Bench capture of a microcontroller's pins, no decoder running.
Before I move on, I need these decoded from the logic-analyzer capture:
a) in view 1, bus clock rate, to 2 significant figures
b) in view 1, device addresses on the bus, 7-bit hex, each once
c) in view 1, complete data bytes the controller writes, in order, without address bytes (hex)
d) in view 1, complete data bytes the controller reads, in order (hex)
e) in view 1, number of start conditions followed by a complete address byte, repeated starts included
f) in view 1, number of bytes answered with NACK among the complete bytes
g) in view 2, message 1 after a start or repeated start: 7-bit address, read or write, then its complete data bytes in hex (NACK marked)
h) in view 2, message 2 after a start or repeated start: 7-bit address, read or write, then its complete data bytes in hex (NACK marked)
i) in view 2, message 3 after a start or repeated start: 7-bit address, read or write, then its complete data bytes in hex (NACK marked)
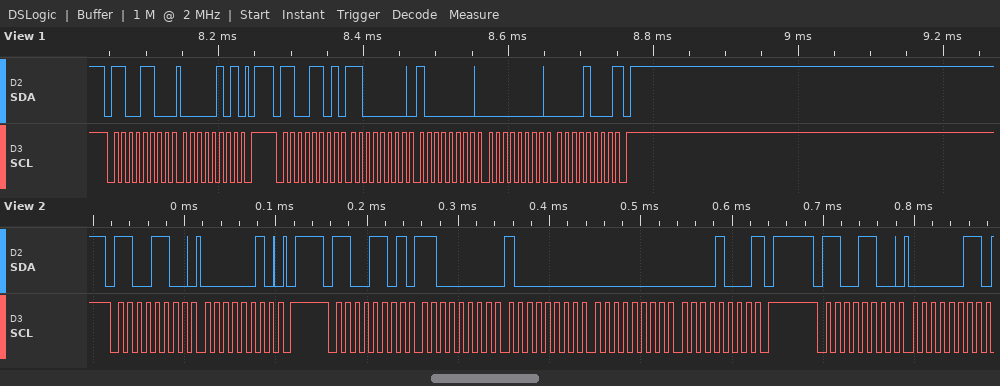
100 kHz
0x66
05
C0 80 00 08
2
1
0x66 write: 02
0x66 read: C0 80 00 08 NACK
0x66 write: 03
